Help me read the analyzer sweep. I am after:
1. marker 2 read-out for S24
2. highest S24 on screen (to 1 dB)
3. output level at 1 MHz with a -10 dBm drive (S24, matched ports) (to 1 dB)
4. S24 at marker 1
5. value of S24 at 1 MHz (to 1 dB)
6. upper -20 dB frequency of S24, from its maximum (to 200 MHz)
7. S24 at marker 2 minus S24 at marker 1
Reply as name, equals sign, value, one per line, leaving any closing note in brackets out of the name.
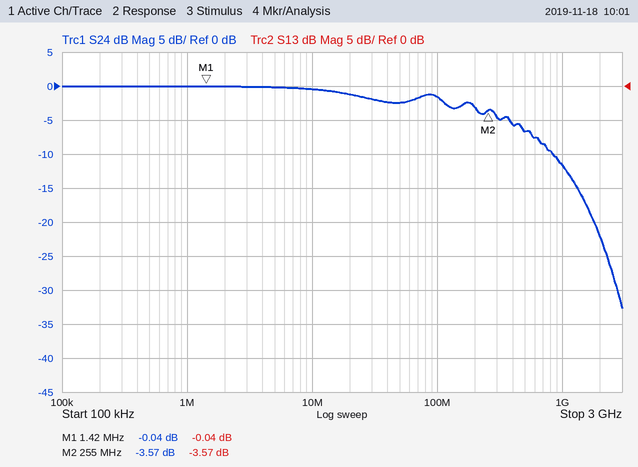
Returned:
marker 2 read-out for S24 = -3.57 dB
highest S24 on screen = 0 dB
output level at 1 MHz with a -10 dBm drive (S24, matched ports) = -10 dBm
S24 at marker 1 = -0.04 dB
value of S24 at 1 MHz = 0 dB
upper -20 dB frequency of S24, from its maximum = 1.8 GHz
S24 at marker 2 minus S24 at marker 1 = -3.53 dB
